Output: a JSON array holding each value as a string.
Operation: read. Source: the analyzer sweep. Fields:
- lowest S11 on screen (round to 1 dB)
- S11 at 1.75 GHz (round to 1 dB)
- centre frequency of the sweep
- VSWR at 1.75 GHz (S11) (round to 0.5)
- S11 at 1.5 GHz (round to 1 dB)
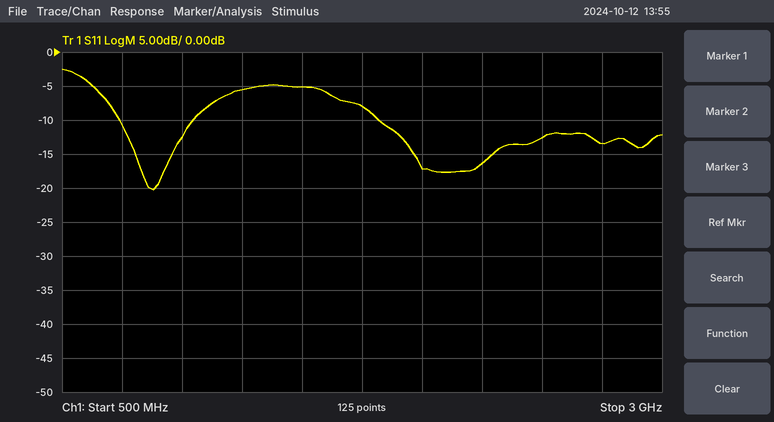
["-20 dB", "-8 dB", "1.75 GHz", "2.5", "-5 dB"]
